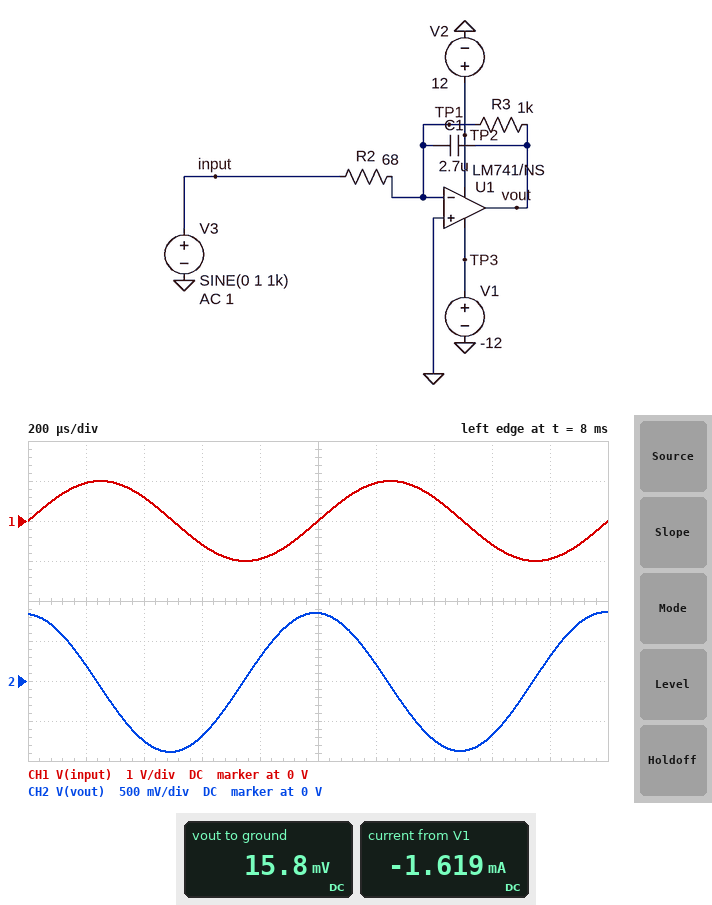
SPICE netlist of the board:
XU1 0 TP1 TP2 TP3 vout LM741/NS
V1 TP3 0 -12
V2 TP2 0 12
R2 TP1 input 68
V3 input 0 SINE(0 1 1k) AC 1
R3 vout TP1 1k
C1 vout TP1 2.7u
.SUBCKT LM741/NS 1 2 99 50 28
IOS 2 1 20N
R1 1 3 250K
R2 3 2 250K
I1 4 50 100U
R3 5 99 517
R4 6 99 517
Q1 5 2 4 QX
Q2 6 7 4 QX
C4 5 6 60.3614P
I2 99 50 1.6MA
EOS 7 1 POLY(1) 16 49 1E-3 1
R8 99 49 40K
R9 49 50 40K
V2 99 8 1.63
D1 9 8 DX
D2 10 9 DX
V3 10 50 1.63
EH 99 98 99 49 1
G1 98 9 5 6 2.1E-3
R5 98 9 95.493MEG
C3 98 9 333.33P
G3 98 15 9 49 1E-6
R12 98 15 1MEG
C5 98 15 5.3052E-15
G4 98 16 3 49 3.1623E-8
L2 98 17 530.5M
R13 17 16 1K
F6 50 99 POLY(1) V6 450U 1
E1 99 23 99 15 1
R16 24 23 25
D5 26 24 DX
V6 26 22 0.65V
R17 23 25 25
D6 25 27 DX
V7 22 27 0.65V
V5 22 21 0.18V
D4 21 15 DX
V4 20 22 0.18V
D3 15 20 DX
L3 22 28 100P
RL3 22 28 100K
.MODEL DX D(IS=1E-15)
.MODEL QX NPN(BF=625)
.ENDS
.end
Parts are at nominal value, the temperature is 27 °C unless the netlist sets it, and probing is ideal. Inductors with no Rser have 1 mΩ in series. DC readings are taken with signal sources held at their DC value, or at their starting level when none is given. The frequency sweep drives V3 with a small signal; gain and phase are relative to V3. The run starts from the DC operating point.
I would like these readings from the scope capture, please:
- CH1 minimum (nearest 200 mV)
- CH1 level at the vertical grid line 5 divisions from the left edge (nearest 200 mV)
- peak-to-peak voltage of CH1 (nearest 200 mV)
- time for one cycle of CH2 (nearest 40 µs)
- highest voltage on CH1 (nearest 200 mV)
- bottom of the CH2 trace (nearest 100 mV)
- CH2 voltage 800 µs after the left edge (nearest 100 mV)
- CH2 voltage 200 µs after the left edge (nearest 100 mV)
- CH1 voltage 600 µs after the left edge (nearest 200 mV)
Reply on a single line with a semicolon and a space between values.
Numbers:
-1.0 V; 0 V; 2.0 V; 1.00 ms; 1.0 V; -900 mV; 300 mV; 200 mV; -600 mV
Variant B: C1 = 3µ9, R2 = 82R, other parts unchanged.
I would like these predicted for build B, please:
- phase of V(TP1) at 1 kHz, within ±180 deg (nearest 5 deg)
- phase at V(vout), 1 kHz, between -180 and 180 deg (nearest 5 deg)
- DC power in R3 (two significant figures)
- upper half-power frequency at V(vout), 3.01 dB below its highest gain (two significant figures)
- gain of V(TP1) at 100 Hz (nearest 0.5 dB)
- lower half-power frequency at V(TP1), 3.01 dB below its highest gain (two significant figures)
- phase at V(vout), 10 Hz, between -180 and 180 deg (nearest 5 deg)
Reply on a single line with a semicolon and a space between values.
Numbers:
75 deg; 90 deg; 150 nW; 41 Hz; -64.5 dB; 320 kHz; 165 deg
